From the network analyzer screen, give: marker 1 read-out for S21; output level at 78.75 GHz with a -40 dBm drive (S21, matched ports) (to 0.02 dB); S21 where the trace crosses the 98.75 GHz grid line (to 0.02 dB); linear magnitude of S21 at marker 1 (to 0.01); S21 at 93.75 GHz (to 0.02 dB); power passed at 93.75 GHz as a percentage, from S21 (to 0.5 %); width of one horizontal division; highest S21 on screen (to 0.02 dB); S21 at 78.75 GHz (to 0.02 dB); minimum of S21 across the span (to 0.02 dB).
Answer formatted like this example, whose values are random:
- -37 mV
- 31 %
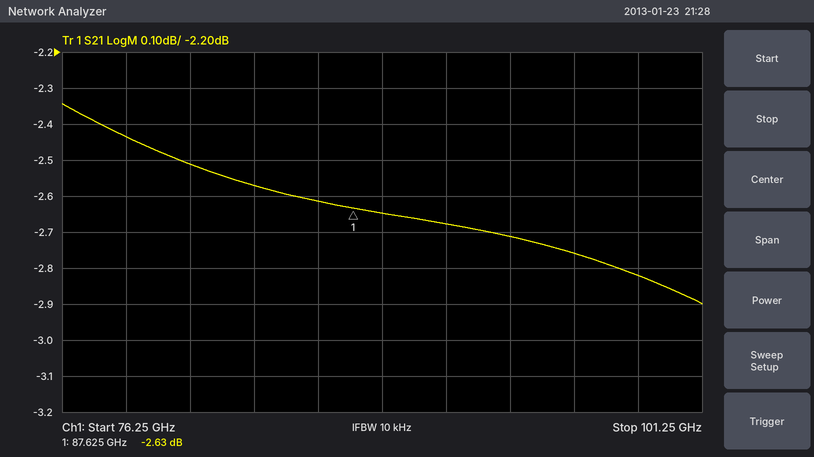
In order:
- -2.63 dB
- -42.44 dBm
- -2.82 dB
- 0.74
- -2.72 dB
- 53.5 %
- 2.5 GHz
- -2.34 dB
- -2.44 dB
- -2.90 dB
